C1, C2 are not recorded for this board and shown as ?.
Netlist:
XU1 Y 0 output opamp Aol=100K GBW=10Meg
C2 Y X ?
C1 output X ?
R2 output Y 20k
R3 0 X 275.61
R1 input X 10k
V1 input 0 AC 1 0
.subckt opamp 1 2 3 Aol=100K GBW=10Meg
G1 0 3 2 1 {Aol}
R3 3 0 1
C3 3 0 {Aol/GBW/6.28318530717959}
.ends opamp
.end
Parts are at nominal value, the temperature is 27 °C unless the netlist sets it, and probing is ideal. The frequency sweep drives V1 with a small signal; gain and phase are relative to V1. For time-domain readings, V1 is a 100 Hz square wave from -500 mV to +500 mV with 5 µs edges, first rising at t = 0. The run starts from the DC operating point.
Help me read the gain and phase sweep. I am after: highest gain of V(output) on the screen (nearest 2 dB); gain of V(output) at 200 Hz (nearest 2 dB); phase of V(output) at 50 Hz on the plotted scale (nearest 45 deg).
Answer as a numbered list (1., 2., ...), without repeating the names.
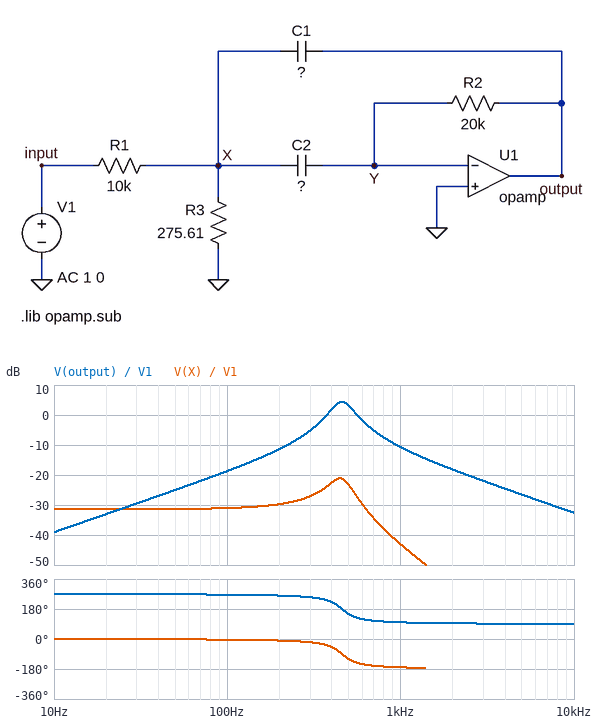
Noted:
1. 4 dB
2. -12 dB
3. 270 deg
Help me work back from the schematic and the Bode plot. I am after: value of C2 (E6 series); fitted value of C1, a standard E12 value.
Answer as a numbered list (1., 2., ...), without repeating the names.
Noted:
1. 330 nF
2. 68 nF
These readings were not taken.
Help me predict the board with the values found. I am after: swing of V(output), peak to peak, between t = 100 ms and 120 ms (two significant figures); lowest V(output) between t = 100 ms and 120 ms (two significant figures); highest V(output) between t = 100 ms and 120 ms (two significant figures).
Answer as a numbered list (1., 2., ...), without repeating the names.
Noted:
1. 810 mV
2. -400 mV
3. 400 mV
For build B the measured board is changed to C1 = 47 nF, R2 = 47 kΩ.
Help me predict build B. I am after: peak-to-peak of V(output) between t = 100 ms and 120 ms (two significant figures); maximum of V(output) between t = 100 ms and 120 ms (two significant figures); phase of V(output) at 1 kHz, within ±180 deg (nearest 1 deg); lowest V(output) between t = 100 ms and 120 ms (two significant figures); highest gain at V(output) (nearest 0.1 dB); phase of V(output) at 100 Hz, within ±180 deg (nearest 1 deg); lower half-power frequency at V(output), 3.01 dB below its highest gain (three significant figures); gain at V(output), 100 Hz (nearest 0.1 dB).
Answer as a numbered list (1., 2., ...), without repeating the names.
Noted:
1. 1.5 V
2. 750 mV
3. 95 deg
4. -750 mV
5. 12.3 dB
6. -94 deg
7. 321 Hz
8. -11.0 dB
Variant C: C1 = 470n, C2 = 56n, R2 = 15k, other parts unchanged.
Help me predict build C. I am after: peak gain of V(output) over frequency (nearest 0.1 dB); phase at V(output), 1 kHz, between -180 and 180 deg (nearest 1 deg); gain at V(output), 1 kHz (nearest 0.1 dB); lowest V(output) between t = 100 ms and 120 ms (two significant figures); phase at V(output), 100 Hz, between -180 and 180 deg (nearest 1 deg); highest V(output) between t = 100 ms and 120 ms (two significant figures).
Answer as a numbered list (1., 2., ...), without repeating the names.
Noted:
1. -15.9 dB
2. 106 deg
3. -27.4 dB
4. -52 mV
5. -95 deg
6. 52 mV
